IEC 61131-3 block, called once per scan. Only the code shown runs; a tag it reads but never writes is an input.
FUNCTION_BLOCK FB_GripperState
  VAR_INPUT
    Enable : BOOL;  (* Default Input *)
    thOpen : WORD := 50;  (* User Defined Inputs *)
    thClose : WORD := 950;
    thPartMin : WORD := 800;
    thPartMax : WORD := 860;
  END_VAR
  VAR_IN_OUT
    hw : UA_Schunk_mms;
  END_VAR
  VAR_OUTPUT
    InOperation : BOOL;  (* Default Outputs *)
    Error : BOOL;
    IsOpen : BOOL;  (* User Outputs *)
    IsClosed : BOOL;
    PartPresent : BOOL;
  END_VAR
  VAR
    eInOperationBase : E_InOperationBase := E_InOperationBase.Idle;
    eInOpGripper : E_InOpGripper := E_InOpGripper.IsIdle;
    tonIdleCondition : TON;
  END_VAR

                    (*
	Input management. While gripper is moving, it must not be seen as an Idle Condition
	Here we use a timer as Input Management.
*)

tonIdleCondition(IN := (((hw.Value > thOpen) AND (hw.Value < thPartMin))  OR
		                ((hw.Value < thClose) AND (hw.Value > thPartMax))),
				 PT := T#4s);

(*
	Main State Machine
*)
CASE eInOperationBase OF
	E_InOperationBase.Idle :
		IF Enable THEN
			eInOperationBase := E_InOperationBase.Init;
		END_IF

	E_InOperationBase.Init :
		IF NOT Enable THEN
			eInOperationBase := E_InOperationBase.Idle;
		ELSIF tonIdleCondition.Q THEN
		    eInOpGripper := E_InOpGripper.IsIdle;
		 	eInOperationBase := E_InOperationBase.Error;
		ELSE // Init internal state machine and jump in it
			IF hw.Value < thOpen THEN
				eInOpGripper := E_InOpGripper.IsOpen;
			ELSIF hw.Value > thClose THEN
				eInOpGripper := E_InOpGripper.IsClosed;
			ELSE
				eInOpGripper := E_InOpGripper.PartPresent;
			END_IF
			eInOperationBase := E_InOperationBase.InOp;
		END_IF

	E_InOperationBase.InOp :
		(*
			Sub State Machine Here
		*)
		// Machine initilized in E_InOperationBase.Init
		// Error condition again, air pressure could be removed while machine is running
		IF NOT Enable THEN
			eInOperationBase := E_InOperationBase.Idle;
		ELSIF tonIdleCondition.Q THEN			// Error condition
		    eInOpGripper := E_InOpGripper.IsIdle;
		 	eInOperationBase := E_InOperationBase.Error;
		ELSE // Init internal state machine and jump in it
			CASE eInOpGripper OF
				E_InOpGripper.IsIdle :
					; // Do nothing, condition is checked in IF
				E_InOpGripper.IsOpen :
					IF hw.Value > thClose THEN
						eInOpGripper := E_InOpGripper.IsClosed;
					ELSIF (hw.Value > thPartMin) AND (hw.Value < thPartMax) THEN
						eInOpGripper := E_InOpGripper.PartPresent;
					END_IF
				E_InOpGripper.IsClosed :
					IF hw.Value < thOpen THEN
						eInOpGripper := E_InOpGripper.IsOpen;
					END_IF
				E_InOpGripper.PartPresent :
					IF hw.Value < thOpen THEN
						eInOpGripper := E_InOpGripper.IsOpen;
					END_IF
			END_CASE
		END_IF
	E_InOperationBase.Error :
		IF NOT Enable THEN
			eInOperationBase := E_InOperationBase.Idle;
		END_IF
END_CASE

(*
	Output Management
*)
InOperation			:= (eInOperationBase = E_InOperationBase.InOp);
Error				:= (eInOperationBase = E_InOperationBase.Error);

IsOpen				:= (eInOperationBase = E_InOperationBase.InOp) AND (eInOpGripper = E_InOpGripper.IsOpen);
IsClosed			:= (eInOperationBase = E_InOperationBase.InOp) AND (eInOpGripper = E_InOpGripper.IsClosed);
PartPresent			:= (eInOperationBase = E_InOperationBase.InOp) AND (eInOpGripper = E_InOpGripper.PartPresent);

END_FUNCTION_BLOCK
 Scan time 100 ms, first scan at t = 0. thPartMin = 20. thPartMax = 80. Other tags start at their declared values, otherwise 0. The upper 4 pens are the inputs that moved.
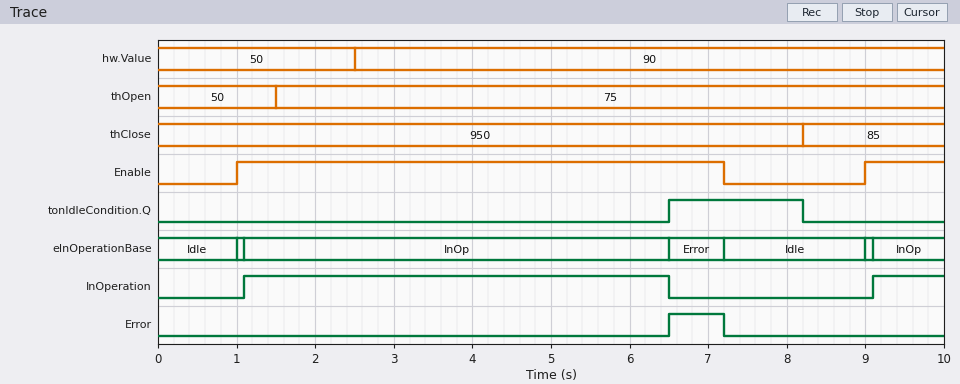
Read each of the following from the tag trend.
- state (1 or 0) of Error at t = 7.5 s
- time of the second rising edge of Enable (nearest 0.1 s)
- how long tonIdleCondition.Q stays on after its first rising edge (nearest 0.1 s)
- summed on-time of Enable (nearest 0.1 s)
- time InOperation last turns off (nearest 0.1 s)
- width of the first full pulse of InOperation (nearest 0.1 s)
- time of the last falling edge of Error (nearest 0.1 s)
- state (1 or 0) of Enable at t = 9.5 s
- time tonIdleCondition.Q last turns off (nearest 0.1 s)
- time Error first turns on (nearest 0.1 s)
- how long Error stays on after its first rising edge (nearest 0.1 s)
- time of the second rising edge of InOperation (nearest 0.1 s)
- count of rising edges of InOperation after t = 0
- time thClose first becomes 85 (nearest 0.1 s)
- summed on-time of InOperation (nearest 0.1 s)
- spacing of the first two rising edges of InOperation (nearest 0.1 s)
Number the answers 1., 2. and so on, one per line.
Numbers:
1. 0
2. 9.0 s
3. 1.7 s
4. 7.2 s
5. 6.5 s
6. 5.4 s
7. 7.2 s
8. 1
9. 8.2 s
10. 6.5 s
11. 0.7 s
12. 9.1 s
13. 2
14. 8.2 s
15. 6.3 s
16. 8.0 s
